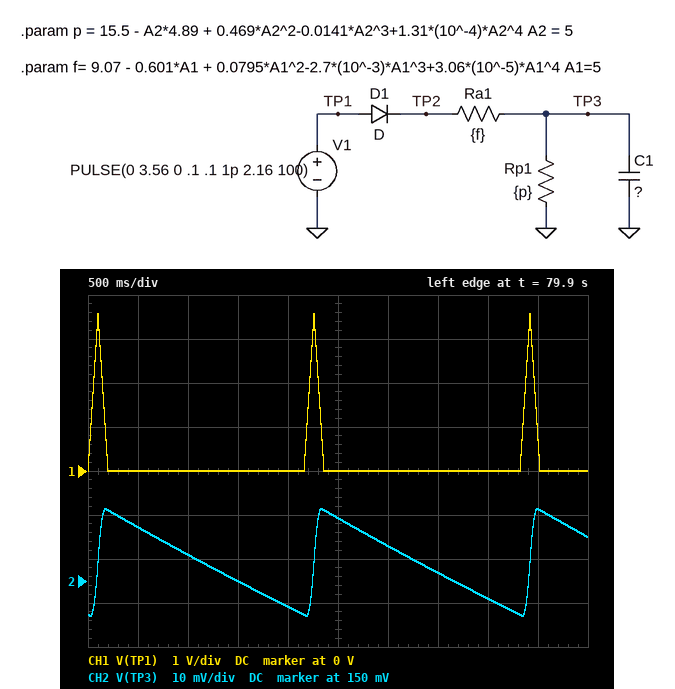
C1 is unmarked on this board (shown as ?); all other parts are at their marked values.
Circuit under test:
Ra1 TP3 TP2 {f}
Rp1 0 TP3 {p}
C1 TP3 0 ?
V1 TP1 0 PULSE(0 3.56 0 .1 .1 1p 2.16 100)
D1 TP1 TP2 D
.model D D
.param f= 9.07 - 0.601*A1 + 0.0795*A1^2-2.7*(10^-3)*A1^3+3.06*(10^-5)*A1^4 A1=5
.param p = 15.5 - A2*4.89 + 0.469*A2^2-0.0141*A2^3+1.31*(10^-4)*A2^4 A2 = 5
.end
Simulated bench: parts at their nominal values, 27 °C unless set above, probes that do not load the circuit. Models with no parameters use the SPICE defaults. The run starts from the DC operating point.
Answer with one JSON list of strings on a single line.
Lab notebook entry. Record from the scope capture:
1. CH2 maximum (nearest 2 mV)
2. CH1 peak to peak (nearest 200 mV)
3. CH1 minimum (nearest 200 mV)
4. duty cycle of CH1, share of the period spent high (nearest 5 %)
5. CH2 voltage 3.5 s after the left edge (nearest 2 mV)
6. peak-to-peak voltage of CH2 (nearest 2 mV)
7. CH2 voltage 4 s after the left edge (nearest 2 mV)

["166 mV", "3.6 V", "0 V", "5 %", "152 mV", "24 mV", "146 mV"]
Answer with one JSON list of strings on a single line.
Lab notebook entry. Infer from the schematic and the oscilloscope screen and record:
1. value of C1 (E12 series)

["820 mF"]
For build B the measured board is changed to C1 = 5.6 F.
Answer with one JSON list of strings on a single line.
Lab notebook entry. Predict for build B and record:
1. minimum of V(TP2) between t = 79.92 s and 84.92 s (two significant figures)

["98 mV"]
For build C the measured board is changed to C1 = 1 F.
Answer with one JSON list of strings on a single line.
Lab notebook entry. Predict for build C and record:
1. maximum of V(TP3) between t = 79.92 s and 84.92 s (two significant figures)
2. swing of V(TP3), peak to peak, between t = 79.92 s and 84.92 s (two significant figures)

["160 mV", "20 mV"]
